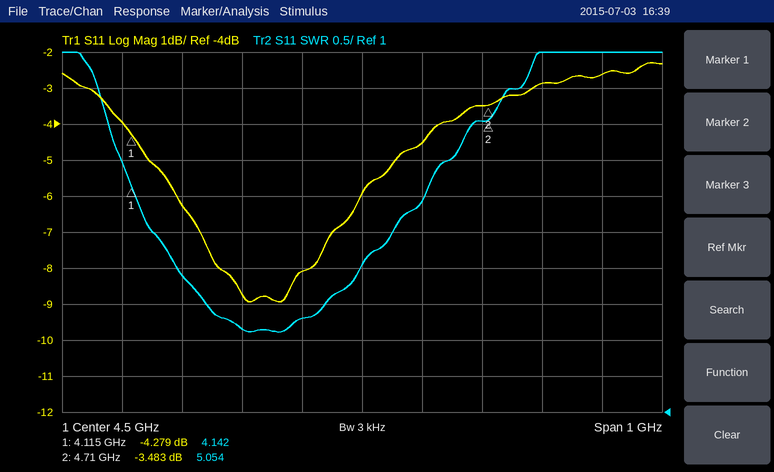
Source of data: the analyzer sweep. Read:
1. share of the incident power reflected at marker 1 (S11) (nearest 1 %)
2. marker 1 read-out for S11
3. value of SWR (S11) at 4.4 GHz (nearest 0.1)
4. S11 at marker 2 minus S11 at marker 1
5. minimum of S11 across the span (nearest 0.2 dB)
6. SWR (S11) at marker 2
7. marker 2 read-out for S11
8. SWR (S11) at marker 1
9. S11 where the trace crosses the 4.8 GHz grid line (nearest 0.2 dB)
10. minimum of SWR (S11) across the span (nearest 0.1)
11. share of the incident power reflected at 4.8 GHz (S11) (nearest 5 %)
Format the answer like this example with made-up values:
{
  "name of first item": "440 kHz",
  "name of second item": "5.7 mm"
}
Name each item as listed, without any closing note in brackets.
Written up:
{
  "share of the incident power reflected at marker 1 (S11)": "37 %",
  "marker 1 read-out for S11": "-4.279 dB",
  "value of SWR (S11) at 4.4 GHz": "2.3",
  "S11 at marker 2 minus S11 at marker 1": "0.796 dB",
  "minimum of S11 across the span": "-9.0 dB",
  "SWR (S11) at marker 2": "5.054",
  "marker 2 read-out for S11": "-3.483 dB",
  "SWR (S11) at marker 1": "4.142",
  "S11 where the trace crosses the 4.8 GHz grid line": "-2.8 dB",
  "minimum of SWR (S11) across the span": "2.1",
  "share of the incident power reflected at 4.8 GHz (S11)": "50 %"
}
